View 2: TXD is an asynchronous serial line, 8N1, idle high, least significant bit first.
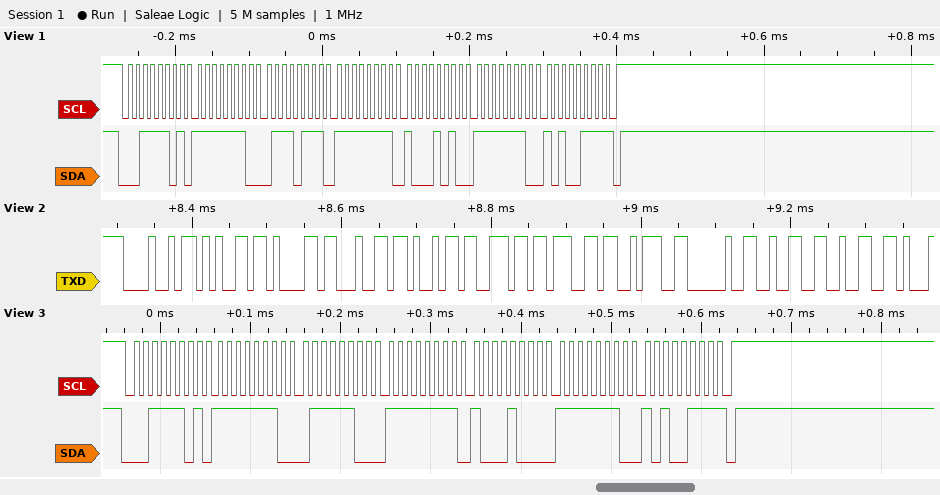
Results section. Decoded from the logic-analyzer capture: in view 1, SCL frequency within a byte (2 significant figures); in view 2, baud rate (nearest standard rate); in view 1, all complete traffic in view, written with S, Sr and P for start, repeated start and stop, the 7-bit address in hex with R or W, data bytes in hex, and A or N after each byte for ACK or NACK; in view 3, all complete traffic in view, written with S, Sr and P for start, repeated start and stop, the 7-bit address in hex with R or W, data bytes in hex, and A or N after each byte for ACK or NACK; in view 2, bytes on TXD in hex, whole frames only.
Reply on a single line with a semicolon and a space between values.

100 kHz; 115200 baud; S 1ER A FE A 77 A FF A 8A A FE A A7 N P; S 1ER A FE A 7C A FF A 88 A FE A A7 N P; 48 65 61 64 69 6E 67 3A 20 32 32
